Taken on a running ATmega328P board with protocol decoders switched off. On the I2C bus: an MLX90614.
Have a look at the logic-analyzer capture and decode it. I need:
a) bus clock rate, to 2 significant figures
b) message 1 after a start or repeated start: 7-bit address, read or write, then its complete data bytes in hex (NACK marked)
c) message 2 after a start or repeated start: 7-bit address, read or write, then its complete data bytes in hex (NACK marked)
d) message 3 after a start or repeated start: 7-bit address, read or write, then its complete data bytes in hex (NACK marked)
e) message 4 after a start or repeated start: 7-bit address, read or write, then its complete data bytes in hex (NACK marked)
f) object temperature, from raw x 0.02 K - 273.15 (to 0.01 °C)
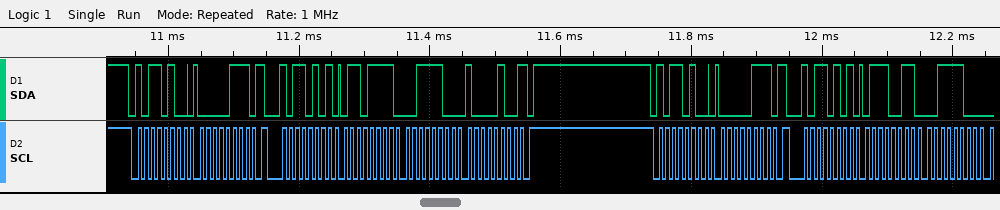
100 kHz
0x5A write: 07
0x5A read: 6F 3C 84 NACK
0x5A write: 07
0x5A read: 73 3C
36.27 °C
